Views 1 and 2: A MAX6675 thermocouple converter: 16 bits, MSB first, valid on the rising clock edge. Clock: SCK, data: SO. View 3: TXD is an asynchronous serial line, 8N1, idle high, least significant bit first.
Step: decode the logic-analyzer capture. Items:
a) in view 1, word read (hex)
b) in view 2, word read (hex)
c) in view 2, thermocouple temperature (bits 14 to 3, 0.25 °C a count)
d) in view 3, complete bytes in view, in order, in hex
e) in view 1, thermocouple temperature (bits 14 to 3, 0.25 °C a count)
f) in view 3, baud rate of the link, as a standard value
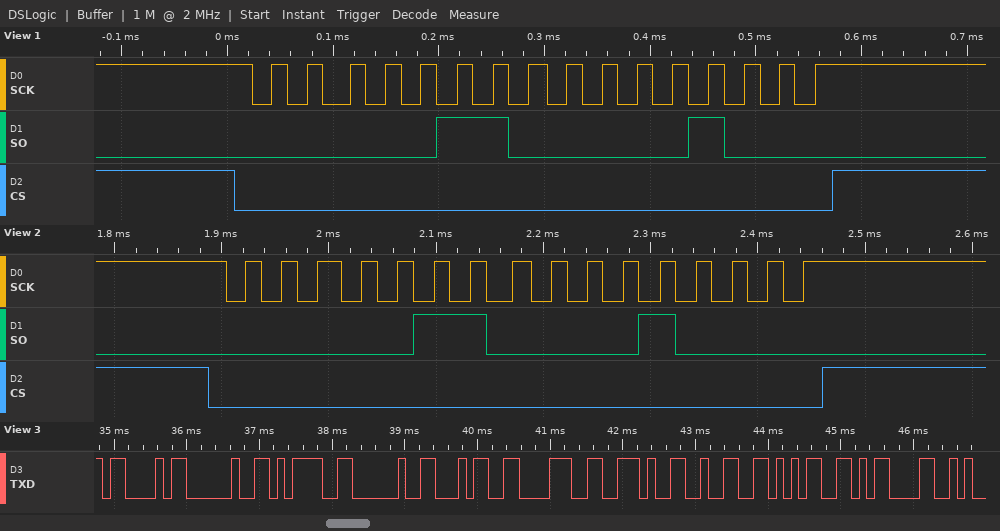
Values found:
0x0608
0x0610
48.50 °C
43 20 3D 20 34 38 2E 32 35 0D
48.25 °C
9600 baud
